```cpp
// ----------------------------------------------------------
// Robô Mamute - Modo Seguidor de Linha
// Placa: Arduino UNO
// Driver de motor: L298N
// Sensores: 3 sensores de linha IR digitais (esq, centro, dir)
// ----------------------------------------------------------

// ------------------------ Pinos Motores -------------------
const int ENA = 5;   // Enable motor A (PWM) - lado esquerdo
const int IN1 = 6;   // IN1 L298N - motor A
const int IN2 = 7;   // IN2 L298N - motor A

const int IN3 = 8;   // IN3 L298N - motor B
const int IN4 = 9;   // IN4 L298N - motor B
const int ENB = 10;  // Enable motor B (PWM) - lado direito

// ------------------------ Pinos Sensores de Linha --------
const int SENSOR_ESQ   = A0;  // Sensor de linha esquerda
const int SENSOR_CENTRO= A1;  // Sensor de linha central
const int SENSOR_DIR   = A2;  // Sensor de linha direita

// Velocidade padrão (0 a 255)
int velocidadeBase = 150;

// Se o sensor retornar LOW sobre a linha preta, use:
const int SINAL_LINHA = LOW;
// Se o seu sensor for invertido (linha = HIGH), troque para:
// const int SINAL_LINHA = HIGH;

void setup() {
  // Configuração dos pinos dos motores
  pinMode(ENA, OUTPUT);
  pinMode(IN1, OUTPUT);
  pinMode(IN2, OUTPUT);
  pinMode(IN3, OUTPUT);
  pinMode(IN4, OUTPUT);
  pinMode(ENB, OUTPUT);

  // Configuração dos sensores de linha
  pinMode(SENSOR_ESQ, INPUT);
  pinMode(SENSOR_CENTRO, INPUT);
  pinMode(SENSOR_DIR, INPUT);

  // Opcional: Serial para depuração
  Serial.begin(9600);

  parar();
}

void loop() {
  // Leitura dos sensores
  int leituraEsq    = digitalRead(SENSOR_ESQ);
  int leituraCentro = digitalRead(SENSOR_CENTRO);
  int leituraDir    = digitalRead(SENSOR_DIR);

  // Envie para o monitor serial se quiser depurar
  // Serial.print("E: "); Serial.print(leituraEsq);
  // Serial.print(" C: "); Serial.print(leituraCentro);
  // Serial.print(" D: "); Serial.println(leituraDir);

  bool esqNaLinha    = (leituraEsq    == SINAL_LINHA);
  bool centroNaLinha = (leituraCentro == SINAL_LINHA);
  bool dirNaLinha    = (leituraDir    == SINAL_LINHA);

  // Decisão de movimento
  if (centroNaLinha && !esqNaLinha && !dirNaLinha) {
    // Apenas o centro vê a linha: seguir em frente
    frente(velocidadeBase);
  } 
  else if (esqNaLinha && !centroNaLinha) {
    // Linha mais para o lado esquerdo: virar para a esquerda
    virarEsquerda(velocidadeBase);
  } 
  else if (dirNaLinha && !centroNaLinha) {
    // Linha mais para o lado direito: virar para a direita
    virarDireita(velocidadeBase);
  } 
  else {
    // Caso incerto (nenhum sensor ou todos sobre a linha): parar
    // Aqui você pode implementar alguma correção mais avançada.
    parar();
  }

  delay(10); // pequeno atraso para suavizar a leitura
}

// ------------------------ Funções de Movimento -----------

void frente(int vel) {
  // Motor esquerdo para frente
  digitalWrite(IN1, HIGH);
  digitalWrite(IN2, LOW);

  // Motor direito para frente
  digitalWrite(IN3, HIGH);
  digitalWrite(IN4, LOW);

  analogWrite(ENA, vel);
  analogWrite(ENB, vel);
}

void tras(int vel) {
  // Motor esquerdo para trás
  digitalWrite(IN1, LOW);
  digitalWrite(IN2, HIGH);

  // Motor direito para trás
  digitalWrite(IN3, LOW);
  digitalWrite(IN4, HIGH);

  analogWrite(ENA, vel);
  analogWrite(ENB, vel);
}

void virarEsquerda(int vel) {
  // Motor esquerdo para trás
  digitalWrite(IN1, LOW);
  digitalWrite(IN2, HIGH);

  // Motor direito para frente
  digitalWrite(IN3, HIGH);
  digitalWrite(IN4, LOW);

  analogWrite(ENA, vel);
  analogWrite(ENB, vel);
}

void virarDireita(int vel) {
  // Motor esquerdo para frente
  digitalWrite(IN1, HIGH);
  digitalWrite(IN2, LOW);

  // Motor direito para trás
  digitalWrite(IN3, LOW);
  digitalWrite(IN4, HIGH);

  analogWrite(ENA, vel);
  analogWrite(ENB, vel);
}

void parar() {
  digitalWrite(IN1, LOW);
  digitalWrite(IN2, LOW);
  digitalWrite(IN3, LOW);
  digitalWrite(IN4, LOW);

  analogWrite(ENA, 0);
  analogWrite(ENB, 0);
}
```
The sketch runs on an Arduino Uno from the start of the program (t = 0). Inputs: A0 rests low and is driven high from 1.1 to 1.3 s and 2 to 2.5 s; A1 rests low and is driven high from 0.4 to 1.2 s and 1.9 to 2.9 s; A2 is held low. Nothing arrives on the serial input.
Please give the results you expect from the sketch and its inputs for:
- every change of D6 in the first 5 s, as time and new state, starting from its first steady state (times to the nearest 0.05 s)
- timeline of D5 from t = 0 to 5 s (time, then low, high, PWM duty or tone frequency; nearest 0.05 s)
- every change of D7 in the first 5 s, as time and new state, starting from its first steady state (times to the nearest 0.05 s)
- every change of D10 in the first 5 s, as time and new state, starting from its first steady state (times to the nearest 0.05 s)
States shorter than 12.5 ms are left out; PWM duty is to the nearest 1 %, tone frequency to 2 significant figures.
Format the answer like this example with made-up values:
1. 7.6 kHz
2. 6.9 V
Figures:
1. 0 s low; 1.1 s high; 1.2 s low; 2 s high; 2.5 s low
2. 0 s low; 0.4 s PWM 59 %; 1.2 s low; 1.9 s PWM 59 %; 2.9 s low
3. 0 s low; 0.4 s high; 1.1 s low; 1.9 s high; 2 s low; 2.5 s high; 2.9 s low
4. 0 s low; 0.4 s PWM 59 %; 1.2 s low; 1.9 s PWM 59 %; 2.9 s low
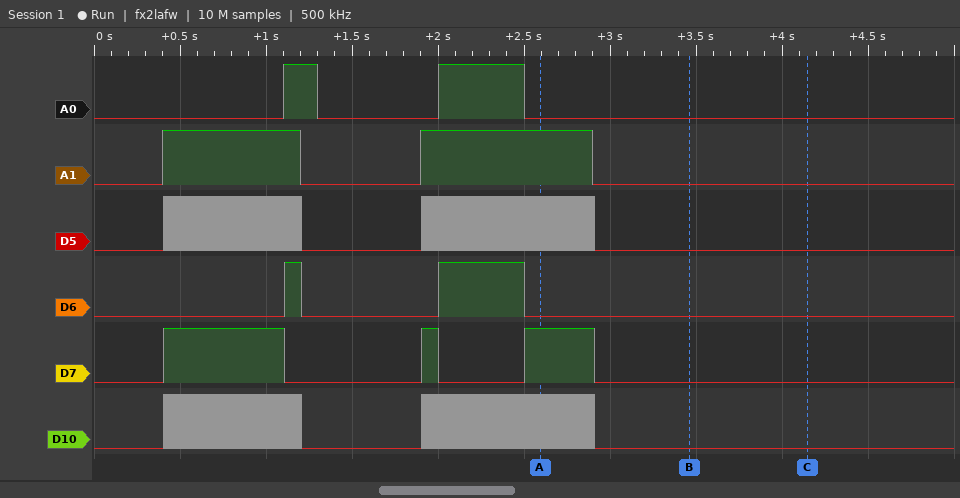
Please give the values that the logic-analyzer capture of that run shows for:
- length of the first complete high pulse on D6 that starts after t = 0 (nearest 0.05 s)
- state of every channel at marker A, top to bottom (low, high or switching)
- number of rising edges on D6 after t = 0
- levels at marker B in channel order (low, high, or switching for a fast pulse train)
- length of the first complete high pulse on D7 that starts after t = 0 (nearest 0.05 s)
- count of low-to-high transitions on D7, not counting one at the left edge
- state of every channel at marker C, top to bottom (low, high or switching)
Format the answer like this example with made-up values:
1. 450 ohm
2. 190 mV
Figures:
1. 0.10 s
2. A0 low, A1 high, D5 switching, D6 low, D7 high, D10 switching
3. 2
4. A0 low, A1 low, D5 low, D6 low, D7 low, D10 low
5. 0.70 s
6. 3
7. A0 low, A1 low, D5 low, D6 low, D7 low, D10 low
